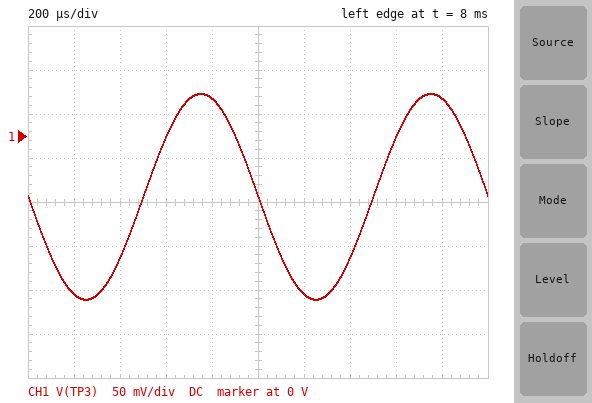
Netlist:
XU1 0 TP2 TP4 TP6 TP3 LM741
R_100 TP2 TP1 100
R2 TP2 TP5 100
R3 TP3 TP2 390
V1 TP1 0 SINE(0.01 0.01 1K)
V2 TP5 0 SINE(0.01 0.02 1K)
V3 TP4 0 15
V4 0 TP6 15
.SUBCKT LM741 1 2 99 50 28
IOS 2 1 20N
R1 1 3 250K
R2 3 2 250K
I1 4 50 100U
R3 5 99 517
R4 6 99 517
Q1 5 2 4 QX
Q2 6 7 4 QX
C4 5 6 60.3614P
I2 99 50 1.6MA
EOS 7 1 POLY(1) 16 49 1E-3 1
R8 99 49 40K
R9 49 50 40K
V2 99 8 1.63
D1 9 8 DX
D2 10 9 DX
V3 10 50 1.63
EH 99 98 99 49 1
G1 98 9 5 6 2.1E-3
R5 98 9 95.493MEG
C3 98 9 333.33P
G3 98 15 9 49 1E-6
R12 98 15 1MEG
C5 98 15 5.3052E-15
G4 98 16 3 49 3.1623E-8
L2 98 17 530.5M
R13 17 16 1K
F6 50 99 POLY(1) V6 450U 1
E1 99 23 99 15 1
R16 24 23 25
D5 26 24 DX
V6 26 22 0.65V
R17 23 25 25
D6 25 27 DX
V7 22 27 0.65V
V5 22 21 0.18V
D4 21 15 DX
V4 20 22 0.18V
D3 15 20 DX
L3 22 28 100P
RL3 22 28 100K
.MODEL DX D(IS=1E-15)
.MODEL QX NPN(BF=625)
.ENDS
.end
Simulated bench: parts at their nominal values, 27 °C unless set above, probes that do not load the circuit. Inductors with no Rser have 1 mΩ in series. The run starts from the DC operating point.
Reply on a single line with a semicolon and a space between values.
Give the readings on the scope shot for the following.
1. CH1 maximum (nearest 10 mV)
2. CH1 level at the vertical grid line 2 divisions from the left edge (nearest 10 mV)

50 mV; -140 mV
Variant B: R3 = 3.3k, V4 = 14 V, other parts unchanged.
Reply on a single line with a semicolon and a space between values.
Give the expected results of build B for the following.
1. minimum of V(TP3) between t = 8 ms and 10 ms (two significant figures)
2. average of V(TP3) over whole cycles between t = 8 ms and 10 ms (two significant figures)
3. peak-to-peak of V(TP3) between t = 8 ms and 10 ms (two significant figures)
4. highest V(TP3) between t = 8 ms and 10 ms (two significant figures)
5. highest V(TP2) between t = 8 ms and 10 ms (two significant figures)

-1.6 V; -590 mV; 2.0 V; 390 mV; 2.0 mV
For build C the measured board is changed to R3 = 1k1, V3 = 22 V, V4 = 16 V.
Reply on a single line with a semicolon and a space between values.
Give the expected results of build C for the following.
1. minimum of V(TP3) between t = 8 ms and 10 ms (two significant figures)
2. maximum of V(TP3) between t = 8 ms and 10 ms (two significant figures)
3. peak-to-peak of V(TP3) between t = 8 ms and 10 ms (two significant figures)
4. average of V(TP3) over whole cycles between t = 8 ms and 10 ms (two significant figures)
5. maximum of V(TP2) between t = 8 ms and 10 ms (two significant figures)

-530 mV; 130 mV; 660 mV; -200 mV; 1.3 mV
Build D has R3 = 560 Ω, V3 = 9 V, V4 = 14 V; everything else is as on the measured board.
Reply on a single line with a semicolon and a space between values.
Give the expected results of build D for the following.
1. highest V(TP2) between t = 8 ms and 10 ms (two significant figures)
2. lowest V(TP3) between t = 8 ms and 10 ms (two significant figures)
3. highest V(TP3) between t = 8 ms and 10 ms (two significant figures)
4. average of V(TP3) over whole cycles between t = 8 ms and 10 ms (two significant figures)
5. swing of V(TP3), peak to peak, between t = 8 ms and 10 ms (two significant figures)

1.3 mV; -270 mV; 69 mV; -99 mV; 340 mV
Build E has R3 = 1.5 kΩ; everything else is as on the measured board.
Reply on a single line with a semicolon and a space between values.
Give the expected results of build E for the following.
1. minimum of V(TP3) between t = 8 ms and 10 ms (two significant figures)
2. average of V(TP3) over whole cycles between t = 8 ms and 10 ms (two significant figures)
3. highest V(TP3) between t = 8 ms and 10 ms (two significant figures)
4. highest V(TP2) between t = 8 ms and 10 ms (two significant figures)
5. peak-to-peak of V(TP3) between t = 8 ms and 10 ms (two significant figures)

-720 mV; -270 mV; 180 mV; 1.5 mV; 900 mV
